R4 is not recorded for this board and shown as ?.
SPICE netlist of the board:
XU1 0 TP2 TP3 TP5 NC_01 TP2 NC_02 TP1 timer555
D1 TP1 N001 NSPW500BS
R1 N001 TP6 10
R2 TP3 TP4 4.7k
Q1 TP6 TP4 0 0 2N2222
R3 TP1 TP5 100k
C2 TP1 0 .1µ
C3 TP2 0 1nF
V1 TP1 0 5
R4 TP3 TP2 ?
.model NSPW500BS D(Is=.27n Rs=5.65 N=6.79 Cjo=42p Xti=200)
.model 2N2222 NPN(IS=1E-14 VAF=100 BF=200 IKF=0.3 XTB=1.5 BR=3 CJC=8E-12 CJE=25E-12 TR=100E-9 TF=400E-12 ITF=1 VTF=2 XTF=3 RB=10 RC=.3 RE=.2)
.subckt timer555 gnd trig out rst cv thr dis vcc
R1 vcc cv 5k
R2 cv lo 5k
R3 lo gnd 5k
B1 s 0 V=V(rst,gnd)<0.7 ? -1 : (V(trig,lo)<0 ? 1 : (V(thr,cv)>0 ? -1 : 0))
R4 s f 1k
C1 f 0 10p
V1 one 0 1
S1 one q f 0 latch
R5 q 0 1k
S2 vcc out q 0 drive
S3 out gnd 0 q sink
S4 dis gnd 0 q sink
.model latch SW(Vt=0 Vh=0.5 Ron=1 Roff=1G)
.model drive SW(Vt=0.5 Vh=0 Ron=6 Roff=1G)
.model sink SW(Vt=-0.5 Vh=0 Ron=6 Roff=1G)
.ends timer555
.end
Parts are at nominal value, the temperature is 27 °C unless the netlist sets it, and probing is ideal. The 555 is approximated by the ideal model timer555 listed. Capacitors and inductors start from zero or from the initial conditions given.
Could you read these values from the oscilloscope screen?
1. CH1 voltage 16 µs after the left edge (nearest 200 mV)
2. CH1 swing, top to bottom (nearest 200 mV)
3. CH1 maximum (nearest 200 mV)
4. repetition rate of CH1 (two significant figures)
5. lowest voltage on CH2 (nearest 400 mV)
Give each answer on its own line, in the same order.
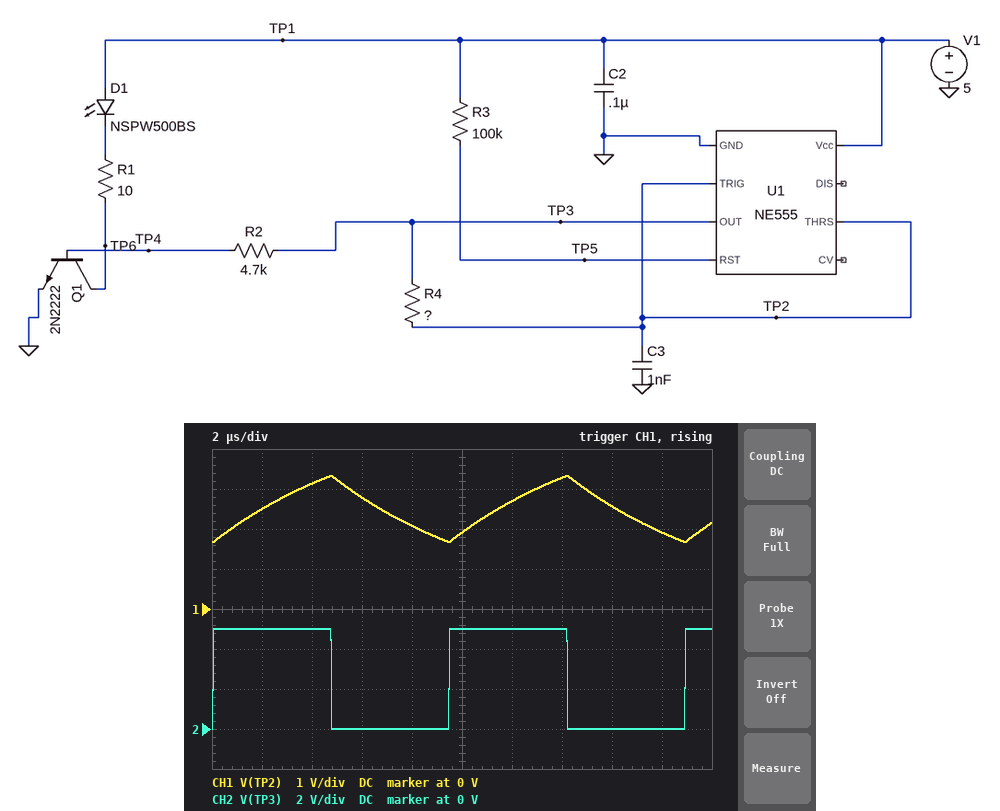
2.6 V
1.6 V
3.4 V
110 kHz
0 V
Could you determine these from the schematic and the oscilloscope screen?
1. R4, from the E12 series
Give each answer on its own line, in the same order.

6.8 kΩ
